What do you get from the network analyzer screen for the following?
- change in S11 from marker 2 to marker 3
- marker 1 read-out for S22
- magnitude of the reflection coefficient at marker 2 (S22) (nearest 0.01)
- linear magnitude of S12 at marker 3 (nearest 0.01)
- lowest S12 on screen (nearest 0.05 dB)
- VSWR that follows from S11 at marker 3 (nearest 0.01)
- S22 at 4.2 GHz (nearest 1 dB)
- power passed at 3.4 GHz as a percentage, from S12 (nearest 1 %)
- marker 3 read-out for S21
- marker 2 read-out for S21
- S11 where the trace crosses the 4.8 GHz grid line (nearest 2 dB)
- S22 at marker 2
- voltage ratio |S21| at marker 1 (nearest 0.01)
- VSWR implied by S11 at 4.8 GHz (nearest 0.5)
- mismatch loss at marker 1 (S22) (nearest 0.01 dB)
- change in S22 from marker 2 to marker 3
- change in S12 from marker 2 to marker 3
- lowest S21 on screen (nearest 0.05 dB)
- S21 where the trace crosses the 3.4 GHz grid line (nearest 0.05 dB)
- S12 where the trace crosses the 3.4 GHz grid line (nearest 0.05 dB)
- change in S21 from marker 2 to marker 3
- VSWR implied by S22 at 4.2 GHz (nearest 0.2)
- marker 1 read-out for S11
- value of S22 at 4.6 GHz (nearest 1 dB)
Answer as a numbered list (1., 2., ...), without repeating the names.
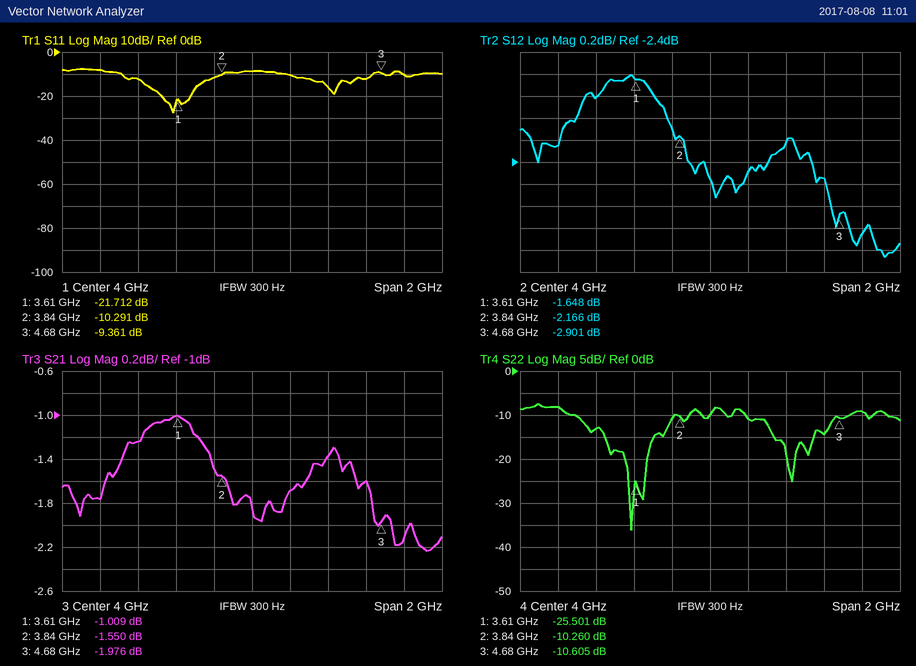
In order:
1. 0.930 dB
2. -25.501 dB
3. 0.31
4. 0.72
5. -3.25 dB
6. 2.03
7. -11 dB
8. 66 %
9. -1.976 dB
10. -1.550 dB
11. -10 dB
12. -10.260 dB
13. 0.89
14. 2.0
15. 0.01 dB
16. -0.345 dB
17. -0.735 dB
18. -2.25 dB
19. -1.25 dB
20. -1.80 dB
21. -0.426 dB
22. 1.8
23. -21.712 dB
24. -14 dB
